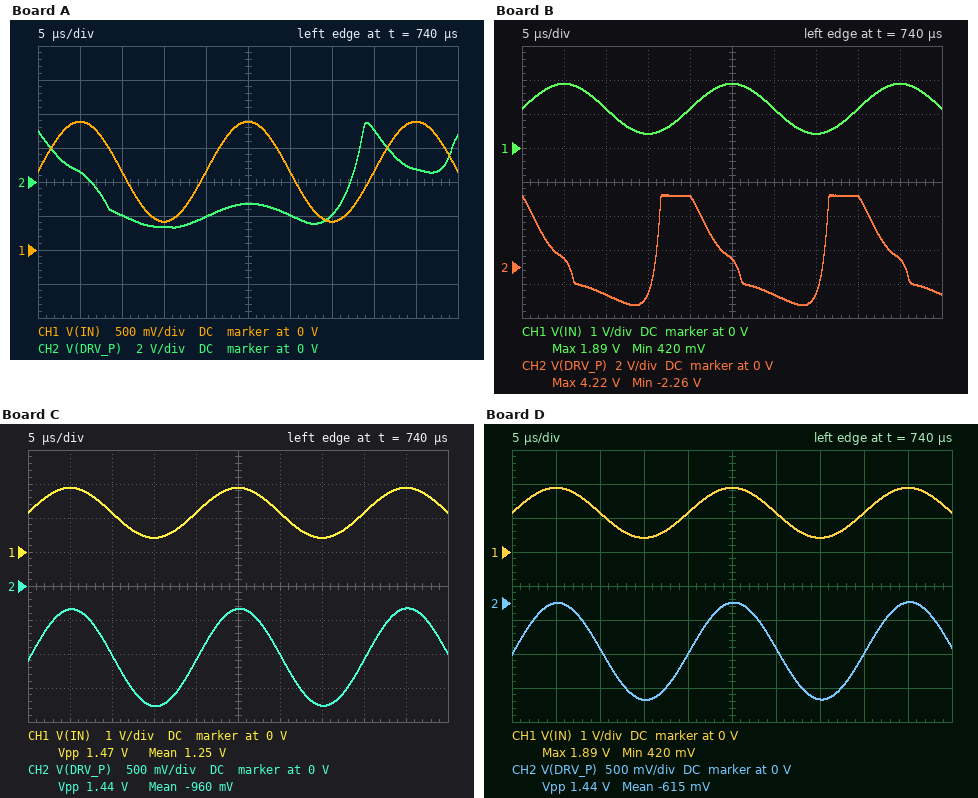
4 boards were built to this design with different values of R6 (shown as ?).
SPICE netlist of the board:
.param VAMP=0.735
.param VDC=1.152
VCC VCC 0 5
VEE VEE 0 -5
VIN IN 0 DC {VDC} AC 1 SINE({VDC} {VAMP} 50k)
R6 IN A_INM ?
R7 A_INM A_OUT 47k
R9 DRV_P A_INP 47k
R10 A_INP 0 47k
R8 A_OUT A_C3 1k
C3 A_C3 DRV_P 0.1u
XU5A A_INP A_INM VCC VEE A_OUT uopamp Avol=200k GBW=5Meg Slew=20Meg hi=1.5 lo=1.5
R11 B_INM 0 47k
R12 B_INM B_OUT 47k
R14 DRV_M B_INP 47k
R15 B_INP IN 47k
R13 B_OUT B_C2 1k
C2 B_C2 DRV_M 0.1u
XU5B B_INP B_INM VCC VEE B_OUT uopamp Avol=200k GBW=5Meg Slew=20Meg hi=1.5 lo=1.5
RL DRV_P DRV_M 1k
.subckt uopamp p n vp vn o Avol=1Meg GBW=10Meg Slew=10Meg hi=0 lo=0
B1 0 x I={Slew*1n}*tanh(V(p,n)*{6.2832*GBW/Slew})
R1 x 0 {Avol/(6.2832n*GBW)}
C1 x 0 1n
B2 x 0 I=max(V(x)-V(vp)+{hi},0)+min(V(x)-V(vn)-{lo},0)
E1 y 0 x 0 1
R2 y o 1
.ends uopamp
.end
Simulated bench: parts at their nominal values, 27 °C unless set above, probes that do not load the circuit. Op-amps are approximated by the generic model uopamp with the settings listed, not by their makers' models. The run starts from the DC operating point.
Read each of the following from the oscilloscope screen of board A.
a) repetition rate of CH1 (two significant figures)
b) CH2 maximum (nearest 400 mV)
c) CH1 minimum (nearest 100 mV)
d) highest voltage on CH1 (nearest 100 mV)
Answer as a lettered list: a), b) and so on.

a) 50 kHz
b) 3.6 V
c) 400 mV
d) 1.9 V
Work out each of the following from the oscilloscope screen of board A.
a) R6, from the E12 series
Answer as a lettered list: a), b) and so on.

a) 39 kΩ
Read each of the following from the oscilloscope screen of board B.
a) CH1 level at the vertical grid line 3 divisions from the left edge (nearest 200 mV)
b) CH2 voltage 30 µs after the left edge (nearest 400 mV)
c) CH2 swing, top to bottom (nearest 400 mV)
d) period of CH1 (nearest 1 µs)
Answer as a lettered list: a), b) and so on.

a) 400 mV
b) -1.6 V
c) 6.4 V
d) 20 µs
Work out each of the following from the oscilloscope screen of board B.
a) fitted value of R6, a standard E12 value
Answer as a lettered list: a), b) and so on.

a) 33 kΩ
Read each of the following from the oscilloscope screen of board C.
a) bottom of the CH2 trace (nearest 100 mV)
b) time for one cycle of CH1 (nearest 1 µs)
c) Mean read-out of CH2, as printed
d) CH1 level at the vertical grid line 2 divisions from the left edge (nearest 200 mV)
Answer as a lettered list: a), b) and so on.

a) -1.8 V
b) 20 µs
c) -960 mV
d) 1.2 V
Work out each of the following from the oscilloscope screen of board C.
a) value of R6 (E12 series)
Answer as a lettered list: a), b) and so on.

a) 22 kΩ
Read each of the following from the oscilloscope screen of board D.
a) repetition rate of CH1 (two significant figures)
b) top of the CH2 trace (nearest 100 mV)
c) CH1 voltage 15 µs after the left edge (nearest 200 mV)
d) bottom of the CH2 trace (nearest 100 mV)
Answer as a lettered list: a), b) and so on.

a) 50 kHz
b) 0 V
c) 400 mV
d) -1.4 V
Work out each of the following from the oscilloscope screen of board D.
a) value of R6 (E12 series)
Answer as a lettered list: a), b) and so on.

a) 18 kΩ
